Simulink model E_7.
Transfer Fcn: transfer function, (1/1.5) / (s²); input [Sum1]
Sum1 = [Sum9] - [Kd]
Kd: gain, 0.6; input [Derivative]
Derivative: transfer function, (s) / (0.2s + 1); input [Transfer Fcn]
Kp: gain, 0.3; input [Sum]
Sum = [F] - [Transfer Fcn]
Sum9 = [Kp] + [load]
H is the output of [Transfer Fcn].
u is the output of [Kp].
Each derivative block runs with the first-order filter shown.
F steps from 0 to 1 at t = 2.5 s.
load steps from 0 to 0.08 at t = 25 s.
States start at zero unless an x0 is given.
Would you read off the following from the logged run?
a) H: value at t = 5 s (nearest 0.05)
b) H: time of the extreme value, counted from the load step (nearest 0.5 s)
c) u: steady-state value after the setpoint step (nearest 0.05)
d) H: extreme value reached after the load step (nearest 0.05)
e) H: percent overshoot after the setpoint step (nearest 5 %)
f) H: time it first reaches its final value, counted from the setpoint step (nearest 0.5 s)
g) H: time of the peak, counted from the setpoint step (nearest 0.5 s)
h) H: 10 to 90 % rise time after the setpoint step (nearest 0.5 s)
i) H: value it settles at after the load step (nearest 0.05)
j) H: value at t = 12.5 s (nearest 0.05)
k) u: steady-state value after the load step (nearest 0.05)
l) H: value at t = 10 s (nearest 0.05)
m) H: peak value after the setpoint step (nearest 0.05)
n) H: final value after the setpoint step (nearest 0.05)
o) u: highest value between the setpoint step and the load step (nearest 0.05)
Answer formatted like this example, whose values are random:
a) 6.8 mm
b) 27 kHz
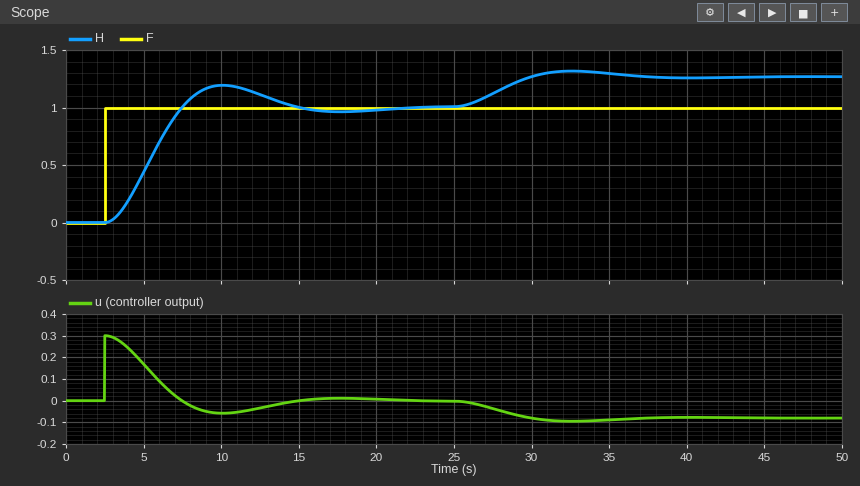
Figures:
a) 0.45
b) 7.5 s
c) 0.00
d) 1.30
e) 20 %
f) 5.0 s
g) 7.5 s
h) 3.5 s
i) 1.25
j) 1.10
k) -0.10
l) 1.20
m) 1.20
n) 1.00
o) 0.30
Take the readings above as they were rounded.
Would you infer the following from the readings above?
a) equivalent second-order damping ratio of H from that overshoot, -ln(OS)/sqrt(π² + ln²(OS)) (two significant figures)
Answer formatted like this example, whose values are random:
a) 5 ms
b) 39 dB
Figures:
a) 0.46
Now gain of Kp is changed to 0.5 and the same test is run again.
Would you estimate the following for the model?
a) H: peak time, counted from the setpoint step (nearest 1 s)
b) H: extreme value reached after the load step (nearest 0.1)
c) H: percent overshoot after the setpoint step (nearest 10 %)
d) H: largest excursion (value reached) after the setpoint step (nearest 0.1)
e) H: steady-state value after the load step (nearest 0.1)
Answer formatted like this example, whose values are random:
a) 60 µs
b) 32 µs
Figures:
a) 6 s
b) 1.2
c) 30 %
d) 1.3
e) 1.2
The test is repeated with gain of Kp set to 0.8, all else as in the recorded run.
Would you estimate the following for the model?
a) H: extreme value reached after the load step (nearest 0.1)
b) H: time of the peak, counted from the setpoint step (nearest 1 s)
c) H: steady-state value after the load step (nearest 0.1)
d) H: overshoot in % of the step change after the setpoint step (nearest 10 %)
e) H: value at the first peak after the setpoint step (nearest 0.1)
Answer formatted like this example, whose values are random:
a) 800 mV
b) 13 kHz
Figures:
a) 1.1
b) 4 s
c) 1.1
d) 40 %
e) 1.4
